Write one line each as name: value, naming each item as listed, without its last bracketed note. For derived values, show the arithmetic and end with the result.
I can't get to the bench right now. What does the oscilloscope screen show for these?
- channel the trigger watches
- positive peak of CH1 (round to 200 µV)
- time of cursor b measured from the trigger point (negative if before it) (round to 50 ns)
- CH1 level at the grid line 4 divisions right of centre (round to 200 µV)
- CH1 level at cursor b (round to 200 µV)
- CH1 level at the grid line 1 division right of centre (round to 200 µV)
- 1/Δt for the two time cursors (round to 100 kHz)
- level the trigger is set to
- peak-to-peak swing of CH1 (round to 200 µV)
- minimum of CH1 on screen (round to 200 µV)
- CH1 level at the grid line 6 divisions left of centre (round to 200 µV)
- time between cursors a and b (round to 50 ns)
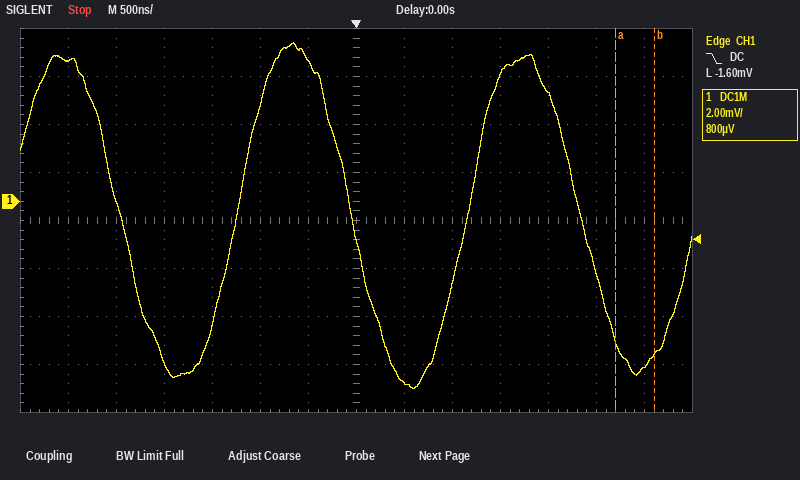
channel the trigger watches: CH1
positive peak of CH1: 6.6 mV
time of cursor b measured from the trigger point (negative if before it): +3.10 µs
CH1 level at the grid line 4 divisions right of centre: 4.6 mV
CH1 level at cursor b: -6.4 mV
CH1 level at the grid line 1 division right of centre: -7.6 mV
1/Δt for the two time cursors: 1 / 400 ns ≈ 2.5 MHz
level the trigger is set to: -1.60 mV
peak-to-peak swing of CH1: 6.6 mV − (-7.8 mV) = 14.4 mV
minimum of CH1 on screen: -7.8 mV
CH1 level at the grid line 6 divisions left of centre: 5.8 mV
time between cursors a and b: 400 ns
